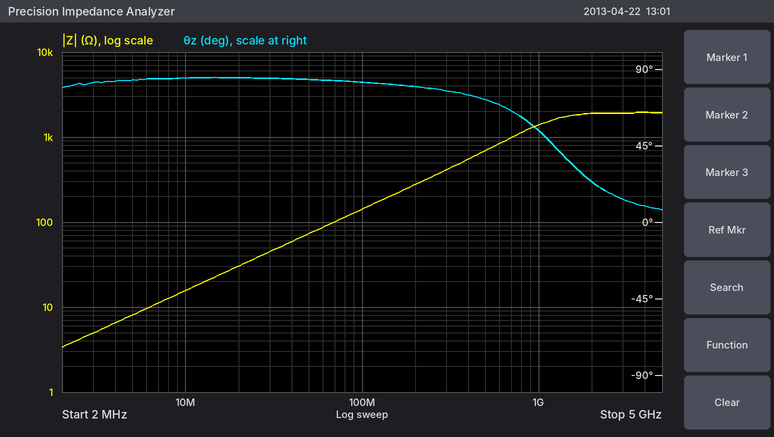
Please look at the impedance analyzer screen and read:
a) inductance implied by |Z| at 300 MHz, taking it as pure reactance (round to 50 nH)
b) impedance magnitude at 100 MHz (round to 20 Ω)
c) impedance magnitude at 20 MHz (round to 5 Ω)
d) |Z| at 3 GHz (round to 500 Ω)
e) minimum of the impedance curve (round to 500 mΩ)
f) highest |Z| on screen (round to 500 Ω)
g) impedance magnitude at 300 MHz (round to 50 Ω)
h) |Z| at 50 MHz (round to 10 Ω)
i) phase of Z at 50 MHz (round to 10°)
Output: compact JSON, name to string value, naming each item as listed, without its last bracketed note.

{"inductance implied by |Z| at 300 MHz, taking it as pure reactance": "200 nH", "impedance magnitude at 100 MHz": "140 Ω", "impedance magnitude at 20 MHz": "30 Ω", "|Z| at 3 GHz": "2.0 kΩ", "minimum of the impedance curve": "3.5 Ω", "highest |Z| on screen": "2.0 kΩ", "impedance magnitude at 300 MHz": "400 Ω", "|Z| at 50 MHz": "70 Ω", "phase of Z at 50 MHz": "80°"}
